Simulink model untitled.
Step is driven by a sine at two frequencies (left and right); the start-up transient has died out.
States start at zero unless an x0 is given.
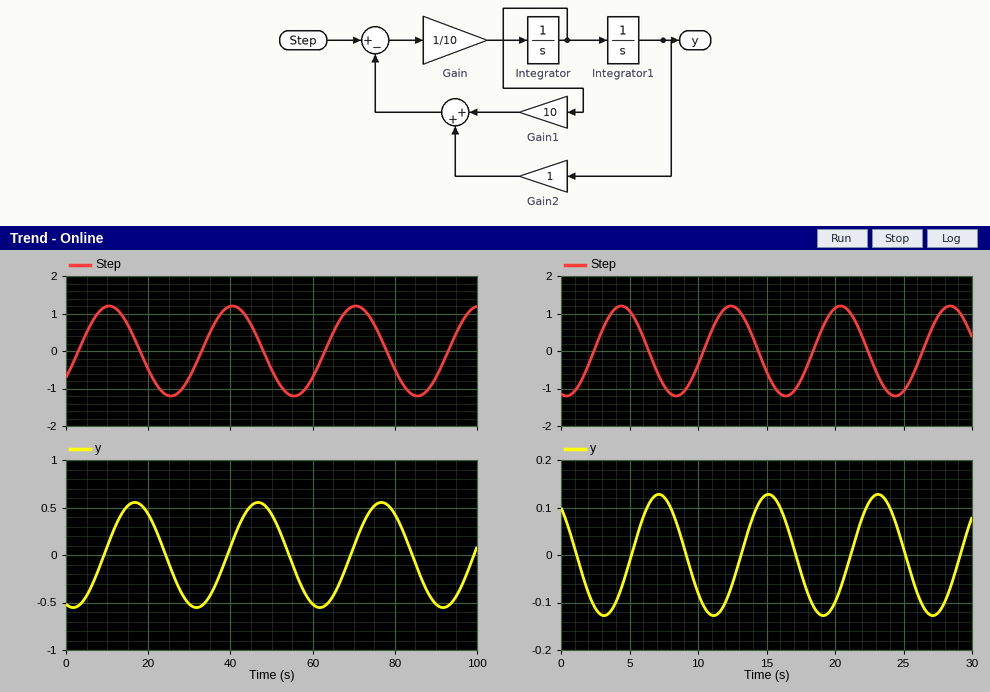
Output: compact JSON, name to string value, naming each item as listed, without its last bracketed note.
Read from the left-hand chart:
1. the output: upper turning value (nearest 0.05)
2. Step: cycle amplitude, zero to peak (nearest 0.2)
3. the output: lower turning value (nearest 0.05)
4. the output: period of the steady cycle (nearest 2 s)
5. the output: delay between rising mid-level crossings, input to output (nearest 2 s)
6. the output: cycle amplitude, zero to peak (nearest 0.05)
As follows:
{"the output: upper turning value": "0.55", "Step: cycle amplitude, zero to peak": "1.2", "the output: lower turning value": "-0.55", "the output: period of the steady cycle": "30 s", "the output: delay between rising mid-level crossings, input to output": "6 s", "the output: cycle amplitude, zero to peak": "0.55"}
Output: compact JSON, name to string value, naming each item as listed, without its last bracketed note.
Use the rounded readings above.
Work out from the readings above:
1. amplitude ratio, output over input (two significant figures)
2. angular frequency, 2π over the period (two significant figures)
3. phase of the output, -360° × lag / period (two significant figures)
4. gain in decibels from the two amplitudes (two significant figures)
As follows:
{"amplitude ratio, output over input": "0.46", "angular frequency, 2π over the period": "0.21 rad/s", "phase of the output, -360° × lag / period": "-72°", "gain in decibels from the two amplitudes": "-6.8 dB"}
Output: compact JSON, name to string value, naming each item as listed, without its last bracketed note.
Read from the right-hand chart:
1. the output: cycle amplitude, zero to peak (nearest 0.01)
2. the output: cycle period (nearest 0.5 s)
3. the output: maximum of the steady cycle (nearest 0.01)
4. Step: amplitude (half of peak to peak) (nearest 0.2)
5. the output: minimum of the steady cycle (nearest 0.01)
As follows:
{"the output: cycle amplitude, zero to peak": "0.13", "the output: cycle period": "8.0 s", "the output: maximum of the steady cycle": "0.13", "Step: amplitude (half of peak to peak)": "1.2", "the output: minimum of the steady cycle": "-0.13"}
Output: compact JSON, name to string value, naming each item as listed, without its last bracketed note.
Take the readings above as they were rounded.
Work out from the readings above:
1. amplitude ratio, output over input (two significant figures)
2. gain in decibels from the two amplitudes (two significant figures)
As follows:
{"amplitude ratio, output over input": "0.11", "gain in decibels from the two amplitudes": "-19 dB"}
